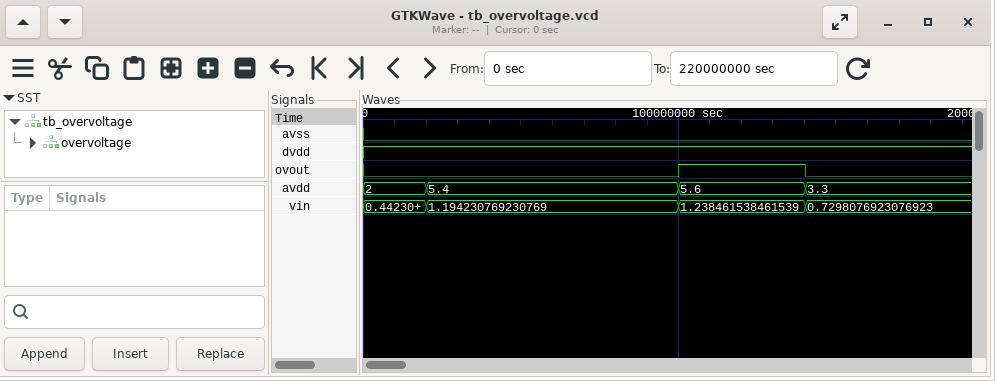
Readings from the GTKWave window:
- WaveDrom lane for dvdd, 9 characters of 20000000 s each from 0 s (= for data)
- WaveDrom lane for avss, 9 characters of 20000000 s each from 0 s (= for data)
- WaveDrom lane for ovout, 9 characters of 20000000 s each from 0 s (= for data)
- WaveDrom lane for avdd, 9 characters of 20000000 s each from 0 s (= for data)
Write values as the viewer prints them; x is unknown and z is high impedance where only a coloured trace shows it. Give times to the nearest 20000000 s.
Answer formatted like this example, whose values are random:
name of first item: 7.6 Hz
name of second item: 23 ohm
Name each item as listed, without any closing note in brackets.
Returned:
WaveDrom lane for dvdd, 9 characters of 20000000 s each from 0 s: {name: 'dvdd', wave: '1........'}
WaveDrom lane for avss, 9 characters of 20000000 s each from 0 s: {name: 'avss', wave: '0........'}
WaveDrom lane for ovout, 9 characters of 20000000 s each from 0 s: {name: 'ovout', wave: '0....1.0.'}
WaveDrom lane for avdd, 9 characters of 20000000 s each from 0 s: {name: 'avdd', wave: '==...=.=.', data: '2 5.4 5.6 3.3'}
